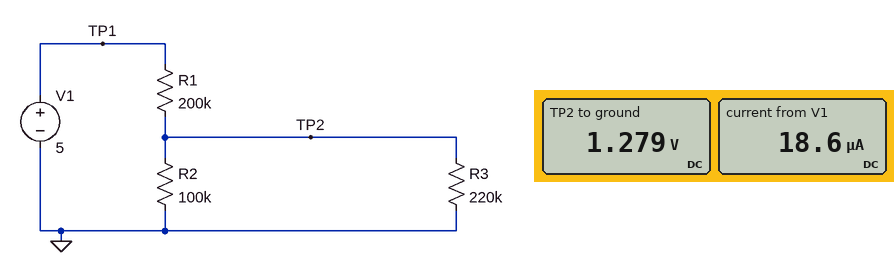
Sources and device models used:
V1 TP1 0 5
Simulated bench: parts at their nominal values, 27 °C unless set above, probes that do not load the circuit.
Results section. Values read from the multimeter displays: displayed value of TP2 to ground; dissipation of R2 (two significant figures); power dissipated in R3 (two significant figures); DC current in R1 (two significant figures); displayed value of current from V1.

1.279 V
16 µW
7.4 µW
19 µA
18.6 µA
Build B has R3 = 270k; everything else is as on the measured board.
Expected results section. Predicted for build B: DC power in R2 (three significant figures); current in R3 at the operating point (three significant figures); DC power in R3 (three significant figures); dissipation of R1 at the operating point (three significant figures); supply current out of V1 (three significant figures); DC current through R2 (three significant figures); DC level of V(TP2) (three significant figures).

17.9 µW
4.95 µA
6.62 µW
67.1 µW
18.3 µA
13.4 µA
1.34 V
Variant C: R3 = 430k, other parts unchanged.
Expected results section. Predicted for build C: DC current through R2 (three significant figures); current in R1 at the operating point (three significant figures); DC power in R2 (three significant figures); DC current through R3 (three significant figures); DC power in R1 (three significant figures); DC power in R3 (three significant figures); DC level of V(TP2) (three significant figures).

14.4 µA
17.8 µA
20.8 µW
3.36 µA
63.3 µW
4.84 µW
1.44 V
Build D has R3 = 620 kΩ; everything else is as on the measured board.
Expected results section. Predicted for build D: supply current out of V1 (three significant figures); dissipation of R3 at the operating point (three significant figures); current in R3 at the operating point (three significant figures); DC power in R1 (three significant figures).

17.5 µA
3.65 µW
2.43 µA
61.1 µW
